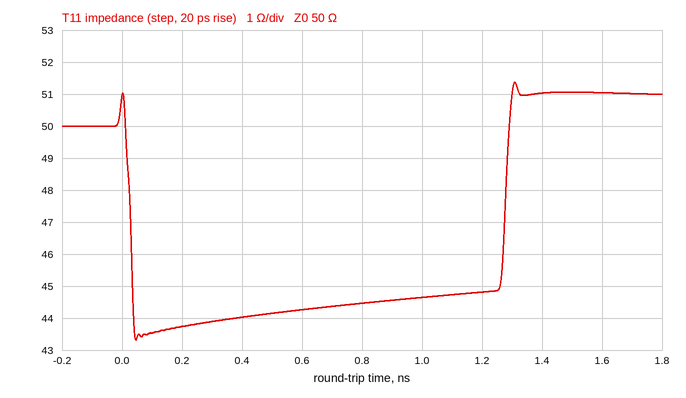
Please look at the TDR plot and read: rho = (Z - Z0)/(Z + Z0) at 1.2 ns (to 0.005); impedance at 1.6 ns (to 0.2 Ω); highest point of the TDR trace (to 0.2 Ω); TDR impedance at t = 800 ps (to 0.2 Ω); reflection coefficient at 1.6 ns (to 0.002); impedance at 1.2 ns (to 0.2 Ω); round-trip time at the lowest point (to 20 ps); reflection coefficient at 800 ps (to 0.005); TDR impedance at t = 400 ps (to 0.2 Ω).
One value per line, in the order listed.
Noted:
-0.055
51.0 Ω
51.4 Ω
44.4 Ω
+0.010
44.8 Ω
40 ps
-0.060
44.0 Ω
